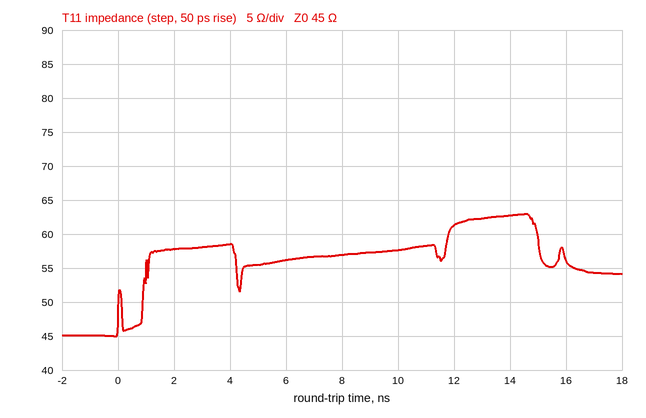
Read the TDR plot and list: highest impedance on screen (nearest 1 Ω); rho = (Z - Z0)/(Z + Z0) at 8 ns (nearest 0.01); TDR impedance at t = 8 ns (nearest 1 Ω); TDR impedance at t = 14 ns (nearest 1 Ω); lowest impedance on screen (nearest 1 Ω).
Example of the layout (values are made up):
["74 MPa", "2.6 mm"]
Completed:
["63 Ω", "+0.12", "57 Ω", "63 Ω", "45 Ω"]
